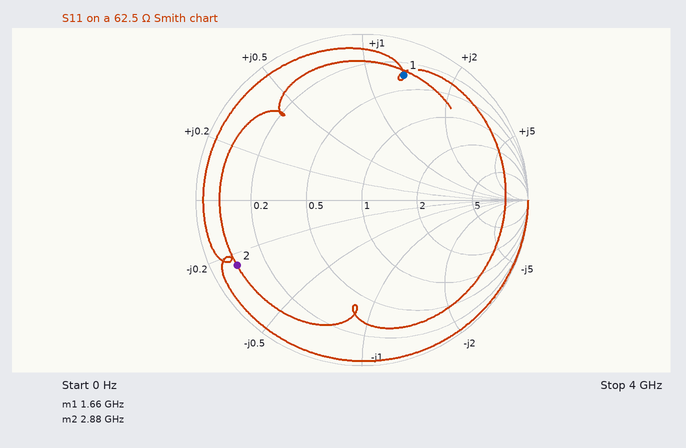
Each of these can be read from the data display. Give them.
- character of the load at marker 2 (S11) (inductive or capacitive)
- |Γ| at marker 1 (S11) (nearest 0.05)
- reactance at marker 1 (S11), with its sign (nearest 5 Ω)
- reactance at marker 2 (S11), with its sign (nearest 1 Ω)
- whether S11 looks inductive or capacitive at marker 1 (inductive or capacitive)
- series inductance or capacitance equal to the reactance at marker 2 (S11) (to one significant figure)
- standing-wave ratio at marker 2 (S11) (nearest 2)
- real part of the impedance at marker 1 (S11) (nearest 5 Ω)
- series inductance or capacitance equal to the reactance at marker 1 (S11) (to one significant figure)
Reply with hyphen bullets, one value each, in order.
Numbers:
- capacitive
- 0.80
- +85 Ω
- -15 Ω
- inductive
- 4 pF
- 12
- 20 Ω
- 8 nH
